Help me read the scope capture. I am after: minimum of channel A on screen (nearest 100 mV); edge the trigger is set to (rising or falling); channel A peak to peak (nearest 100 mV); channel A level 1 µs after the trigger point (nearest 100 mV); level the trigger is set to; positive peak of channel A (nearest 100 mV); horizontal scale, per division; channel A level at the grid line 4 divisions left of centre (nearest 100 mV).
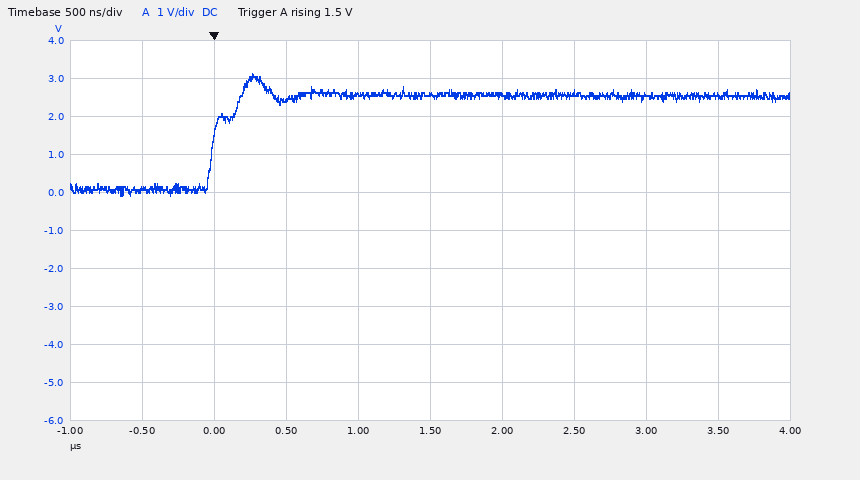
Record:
-100 mV
rising
3.2 V
2.6 V
1.5 V
3.1 V
500 ns
100 mV
